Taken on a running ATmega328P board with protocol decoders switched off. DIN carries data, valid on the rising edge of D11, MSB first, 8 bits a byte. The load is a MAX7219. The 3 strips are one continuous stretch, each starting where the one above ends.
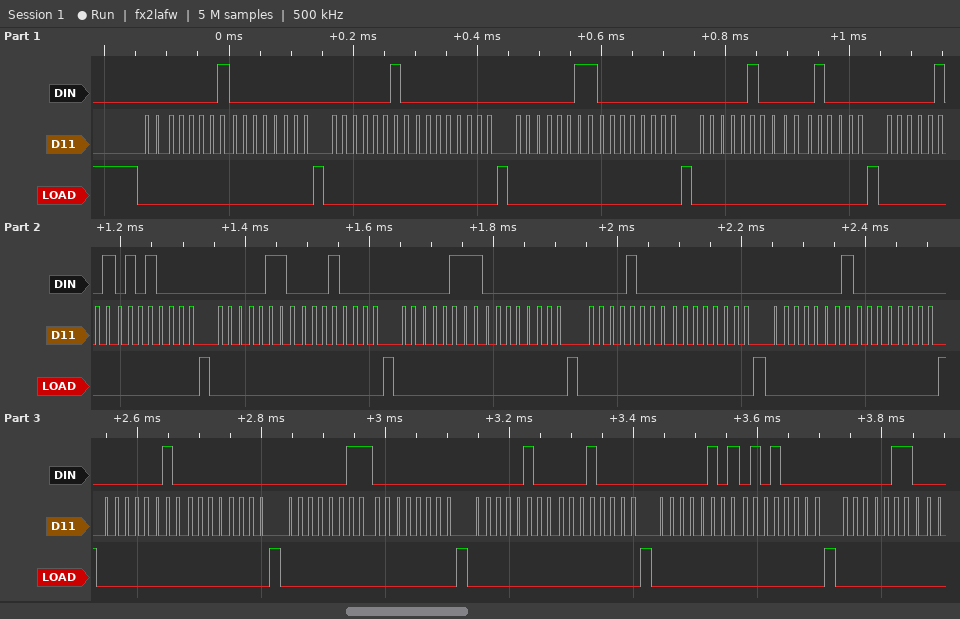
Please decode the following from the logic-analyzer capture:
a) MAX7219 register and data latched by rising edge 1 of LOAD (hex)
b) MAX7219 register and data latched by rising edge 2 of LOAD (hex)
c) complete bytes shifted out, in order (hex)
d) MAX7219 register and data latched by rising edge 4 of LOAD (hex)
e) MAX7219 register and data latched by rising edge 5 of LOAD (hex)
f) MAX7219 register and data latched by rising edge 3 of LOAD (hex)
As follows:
register 0x1, data 0x00
register 0x2, data 0x00
01 00 02 00 03 00 04 10 05 50 06 10 07 00 08 00 01 00 02 00 03 00 04 10 05 50 06
register 0x4, data 0x10
register 0x5, data 0x50
register 0x3, data 0x00
